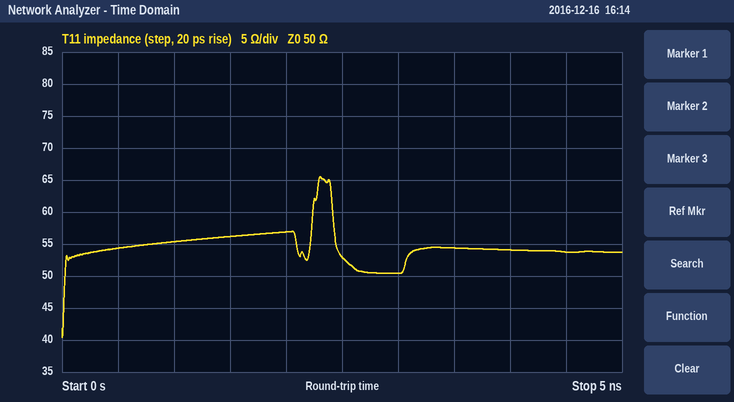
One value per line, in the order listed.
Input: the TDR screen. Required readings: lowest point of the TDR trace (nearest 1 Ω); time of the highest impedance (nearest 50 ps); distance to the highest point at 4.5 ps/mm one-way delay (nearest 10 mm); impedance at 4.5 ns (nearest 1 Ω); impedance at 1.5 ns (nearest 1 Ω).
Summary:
40 Ω
2.30 ns
260 mm
54 Ω
56 Ω
